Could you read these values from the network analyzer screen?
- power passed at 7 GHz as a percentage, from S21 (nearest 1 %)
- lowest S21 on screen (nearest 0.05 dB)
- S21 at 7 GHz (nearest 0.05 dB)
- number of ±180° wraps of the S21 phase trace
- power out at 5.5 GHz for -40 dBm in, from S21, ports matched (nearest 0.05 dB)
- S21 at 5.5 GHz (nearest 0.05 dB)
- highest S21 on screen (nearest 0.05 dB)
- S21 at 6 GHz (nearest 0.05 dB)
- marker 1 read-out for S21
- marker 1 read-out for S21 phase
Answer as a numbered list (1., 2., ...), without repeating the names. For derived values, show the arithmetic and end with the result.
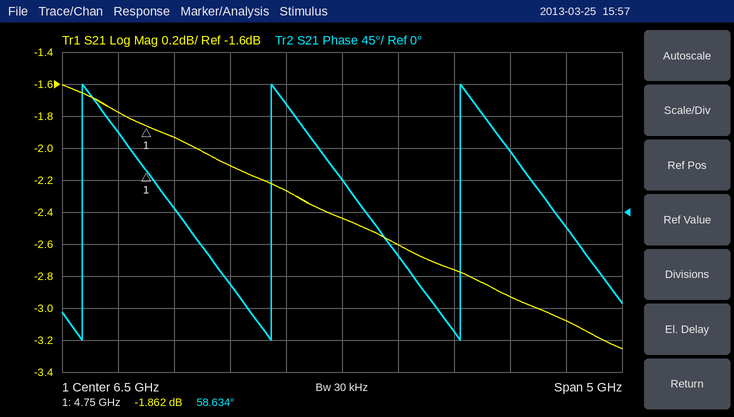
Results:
1. 10^(-2.6/10) ≈ 55 %
2. -3.25 dB
3. -2.60 dB
4. 3
5. -40 dBm + (-2.10 dB) = -42.10 dBm
6. -2.10 dB
7. -1.60 dB
8. -2.25 dB
9. -1.862 dB
10. 58.634°
